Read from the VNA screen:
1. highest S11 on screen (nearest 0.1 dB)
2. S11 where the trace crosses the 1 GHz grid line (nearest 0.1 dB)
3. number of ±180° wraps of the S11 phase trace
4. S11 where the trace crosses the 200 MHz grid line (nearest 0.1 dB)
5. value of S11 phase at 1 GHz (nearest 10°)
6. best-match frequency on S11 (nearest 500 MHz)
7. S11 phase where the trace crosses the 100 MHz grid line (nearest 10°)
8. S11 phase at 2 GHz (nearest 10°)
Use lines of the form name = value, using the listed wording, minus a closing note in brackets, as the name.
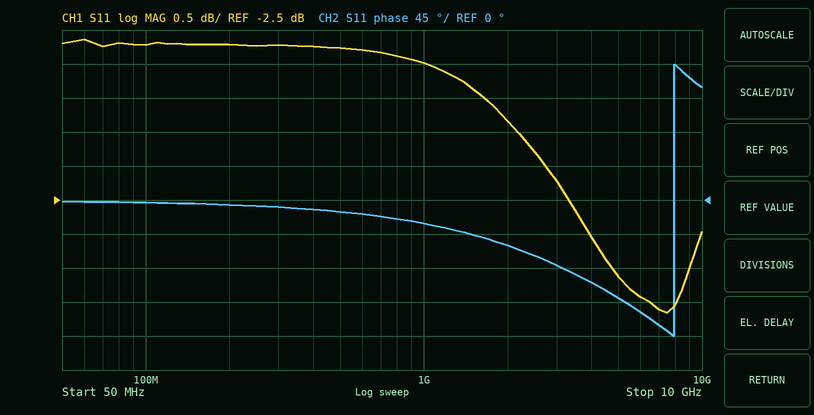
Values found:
highest S11 on screen = -0.1 dB
S11 where the trace crosses the 1 GHz grid line = -0.5 dB
number of ±180° wraps of the S11 phase trace = 1
S11 where the trace crosses the 200 MHz grid line = -0.2 dB
value of S11 phase at 1 GHz = -30°
best-match frequency on S11 = 7.5 GHz
S11 phase where the trace crosses the 100 MHz grid line = 0°
S11 phase at 2 GHz = -60°
